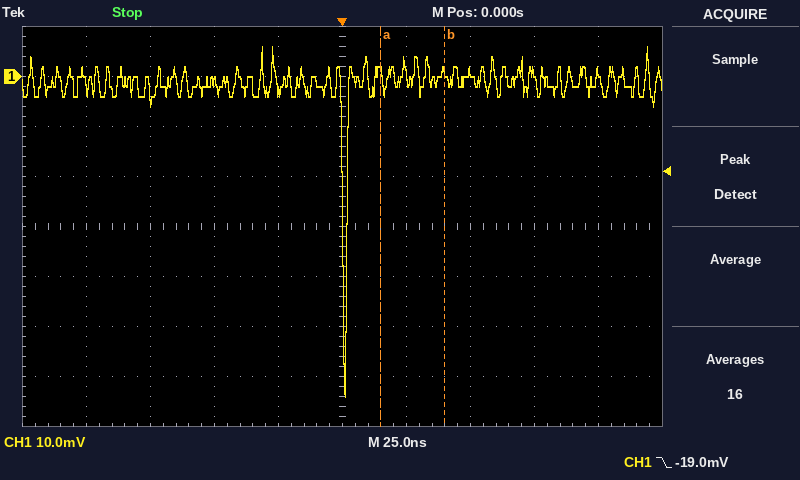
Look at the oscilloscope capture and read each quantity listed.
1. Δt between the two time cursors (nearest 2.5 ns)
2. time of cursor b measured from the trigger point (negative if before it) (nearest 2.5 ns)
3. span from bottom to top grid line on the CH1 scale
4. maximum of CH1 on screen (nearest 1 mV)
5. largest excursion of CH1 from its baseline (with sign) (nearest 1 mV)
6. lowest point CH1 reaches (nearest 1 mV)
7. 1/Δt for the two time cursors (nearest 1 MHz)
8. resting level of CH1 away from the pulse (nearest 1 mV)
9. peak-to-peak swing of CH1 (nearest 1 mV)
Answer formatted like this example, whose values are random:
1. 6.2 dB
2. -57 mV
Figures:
1. 25.0 ns
2. +40.0 ns
3. 80 mV
4. 6 mV
5. -63 mV
6. -64 mV
7. 40 MHz
8. -1 mV
9. 70 mV
